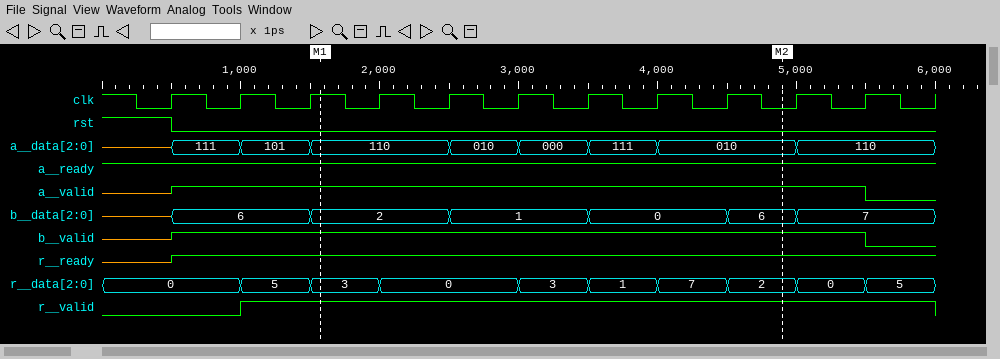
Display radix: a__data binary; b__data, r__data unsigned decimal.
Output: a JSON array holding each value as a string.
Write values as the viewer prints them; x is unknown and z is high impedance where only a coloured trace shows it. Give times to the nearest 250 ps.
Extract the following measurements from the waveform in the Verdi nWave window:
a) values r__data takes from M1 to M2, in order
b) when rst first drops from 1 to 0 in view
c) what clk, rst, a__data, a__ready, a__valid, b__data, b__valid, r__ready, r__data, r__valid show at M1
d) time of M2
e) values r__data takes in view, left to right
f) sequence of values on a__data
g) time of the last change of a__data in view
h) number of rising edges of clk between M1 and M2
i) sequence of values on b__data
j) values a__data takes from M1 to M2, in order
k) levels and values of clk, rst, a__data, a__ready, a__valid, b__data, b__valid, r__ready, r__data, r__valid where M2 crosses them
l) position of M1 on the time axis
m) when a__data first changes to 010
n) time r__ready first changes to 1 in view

["3, 0, 3, 1, 7, 2", "500 ps", "clk=1, rst=0, a__data=110, a__ready=1, a__valid=1, b__data=2, b__valid=1, r__ready=1, r__data=3, r__valid=1", "5000 ps", "0, 5, 3, 0, 3, 1, 7, 2, 0, 5", "z, 111, 101, 110, 010, 000, 111, 010, 110", "5000 ps", "6", "z, 6, 2, 1, 0, 6, 7", "110, 010, 000, 111, 010", "clk=0, rst=0, a__data=010, a__ready=1, a__valid=1, b__data=6, b__valid=1, r__ready=1, r__data=2, r__valid=1", "1500 ps", "2500 ps", "500 ps"]
